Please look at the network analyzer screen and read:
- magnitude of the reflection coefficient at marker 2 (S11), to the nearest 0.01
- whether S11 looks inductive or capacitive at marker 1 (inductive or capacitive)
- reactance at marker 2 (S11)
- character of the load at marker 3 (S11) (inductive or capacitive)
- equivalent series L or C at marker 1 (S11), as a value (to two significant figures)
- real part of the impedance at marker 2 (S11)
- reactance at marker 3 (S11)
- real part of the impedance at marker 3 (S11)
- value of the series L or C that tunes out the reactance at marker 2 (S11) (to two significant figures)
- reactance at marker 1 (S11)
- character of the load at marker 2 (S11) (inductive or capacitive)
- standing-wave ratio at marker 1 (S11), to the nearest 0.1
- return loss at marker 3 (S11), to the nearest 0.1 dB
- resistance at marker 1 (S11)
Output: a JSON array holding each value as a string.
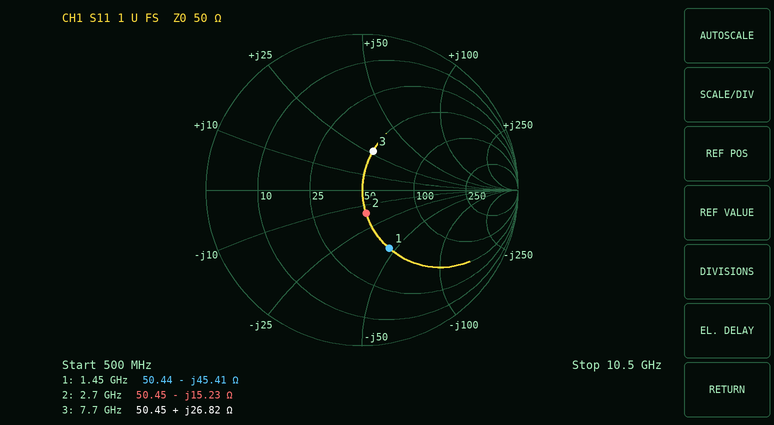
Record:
["0.15", "capacitive", "-15.23 Ω", "inductive", "2.4 pF", "50.45 Ω", "+26.82 Ω", "50.45 Ω", "900 pH", "-45.41 Ω", "capacitive", "2.4", "11.8 dB", "50.44 Ω"]
